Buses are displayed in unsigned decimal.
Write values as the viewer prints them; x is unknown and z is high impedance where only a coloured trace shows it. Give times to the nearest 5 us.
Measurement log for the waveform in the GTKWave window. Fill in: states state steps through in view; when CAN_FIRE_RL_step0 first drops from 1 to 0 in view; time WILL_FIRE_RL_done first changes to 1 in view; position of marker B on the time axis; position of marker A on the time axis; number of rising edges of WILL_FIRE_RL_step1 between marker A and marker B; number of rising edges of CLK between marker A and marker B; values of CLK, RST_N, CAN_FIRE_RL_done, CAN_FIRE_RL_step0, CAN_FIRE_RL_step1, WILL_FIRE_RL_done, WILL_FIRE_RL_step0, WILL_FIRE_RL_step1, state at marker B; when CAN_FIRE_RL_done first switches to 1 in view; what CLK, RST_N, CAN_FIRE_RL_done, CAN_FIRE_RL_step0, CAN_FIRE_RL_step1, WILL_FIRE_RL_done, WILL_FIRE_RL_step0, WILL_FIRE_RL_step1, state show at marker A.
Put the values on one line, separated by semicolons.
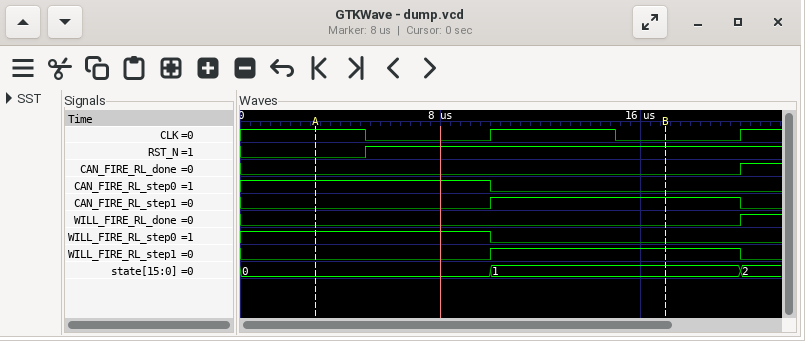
0, 1, 2; 10 us; 20 us; 15 us; 5 us; 1; 1; CLK=0, RST_N=1, CAN_FIRE_RL_done=0, CAN_FIRE_RL_step0=0, CAN_FIRE_RL_step1=1, WILL_FIRE_RL_done=0, WILL_FIRE_RL_step0=0, WILL_FIRE_RL_step1=1, state=1; 20 us; CLK=1, RST_N=0, CAN_FIRE_RL_done=0, CAN_FIRE_RL_step0=1, CAN_FIRE_RL_step1=0, WILL_FIRE_RL_done=0, WILL_FIRE_RL_step0=1, WILL_FIRE_RL_step1=0, state=0
